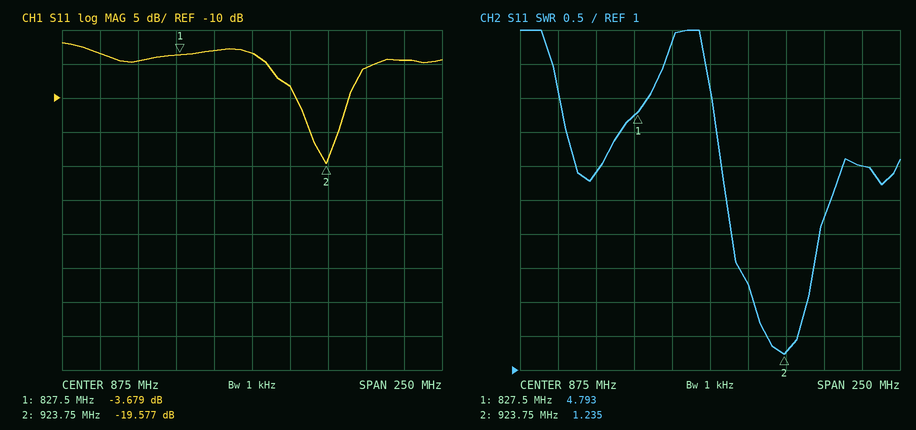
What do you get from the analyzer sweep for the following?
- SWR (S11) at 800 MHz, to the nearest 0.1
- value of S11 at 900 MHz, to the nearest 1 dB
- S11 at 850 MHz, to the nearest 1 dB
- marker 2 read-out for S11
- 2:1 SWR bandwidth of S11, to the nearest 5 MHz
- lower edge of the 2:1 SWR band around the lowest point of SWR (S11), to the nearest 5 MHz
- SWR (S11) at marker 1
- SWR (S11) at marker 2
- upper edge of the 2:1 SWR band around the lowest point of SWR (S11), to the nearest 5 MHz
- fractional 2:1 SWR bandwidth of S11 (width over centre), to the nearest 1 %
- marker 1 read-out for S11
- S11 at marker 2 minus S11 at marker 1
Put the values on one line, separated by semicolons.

3.9; -8 dB; -3 dB; -19.577 dB; 35 MHz; 905 MHz; 4.793; 1.235; 940 MHz; 4 %; -3.679 dB; -15.898 dB
